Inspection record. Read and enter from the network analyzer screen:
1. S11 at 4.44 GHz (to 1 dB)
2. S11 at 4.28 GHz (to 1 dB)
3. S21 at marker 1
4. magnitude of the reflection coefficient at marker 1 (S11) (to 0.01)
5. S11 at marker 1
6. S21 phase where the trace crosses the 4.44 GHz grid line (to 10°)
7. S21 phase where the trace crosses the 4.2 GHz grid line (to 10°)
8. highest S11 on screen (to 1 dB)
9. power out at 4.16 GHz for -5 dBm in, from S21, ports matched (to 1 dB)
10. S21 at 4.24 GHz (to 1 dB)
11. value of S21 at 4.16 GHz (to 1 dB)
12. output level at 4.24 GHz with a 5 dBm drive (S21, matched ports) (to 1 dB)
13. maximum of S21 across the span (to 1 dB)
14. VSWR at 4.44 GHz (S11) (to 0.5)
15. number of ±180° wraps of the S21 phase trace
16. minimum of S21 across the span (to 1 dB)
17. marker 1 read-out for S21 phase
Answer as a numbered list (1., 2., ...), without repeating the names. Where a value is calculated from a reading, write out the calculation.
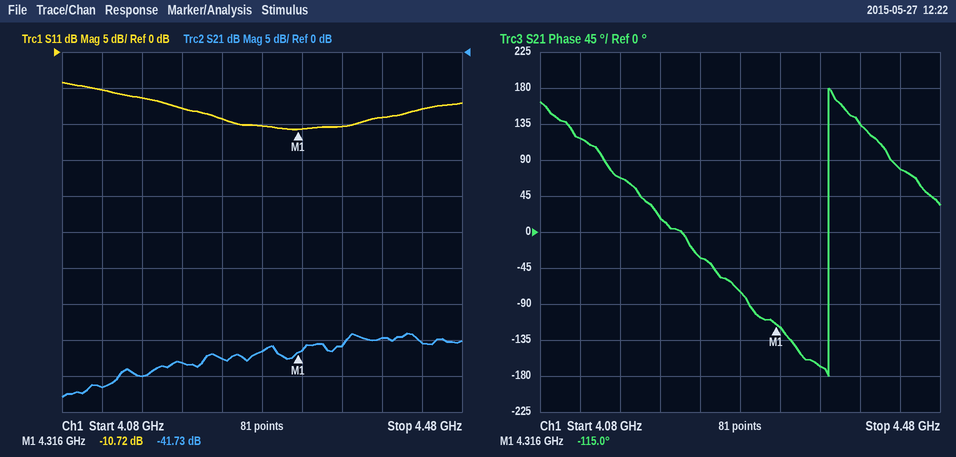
1. -8 dB
2. -10 dB
3. -41.73 dB
4. 10^(-10.72/20) ≈ 0.29
5. -10.72 dB
6. 80°
7. 20°
8. -4 dB
9. -5 dBm + (-45 dB) = -50 dBm
10. -43 dB
11. -45 dB
12. 5 dBm + (-43 dB) = -38 dBm
13. -39 dB
14. |Γ| = 10^(-8/20) = 0.3981; VSWR = (1 + 0.3981)/(1 − 0.3981) ≈ 2.32, so 2.5 to the nearest 0.5
15. 1
16. -48 dB
17. -115.0°
